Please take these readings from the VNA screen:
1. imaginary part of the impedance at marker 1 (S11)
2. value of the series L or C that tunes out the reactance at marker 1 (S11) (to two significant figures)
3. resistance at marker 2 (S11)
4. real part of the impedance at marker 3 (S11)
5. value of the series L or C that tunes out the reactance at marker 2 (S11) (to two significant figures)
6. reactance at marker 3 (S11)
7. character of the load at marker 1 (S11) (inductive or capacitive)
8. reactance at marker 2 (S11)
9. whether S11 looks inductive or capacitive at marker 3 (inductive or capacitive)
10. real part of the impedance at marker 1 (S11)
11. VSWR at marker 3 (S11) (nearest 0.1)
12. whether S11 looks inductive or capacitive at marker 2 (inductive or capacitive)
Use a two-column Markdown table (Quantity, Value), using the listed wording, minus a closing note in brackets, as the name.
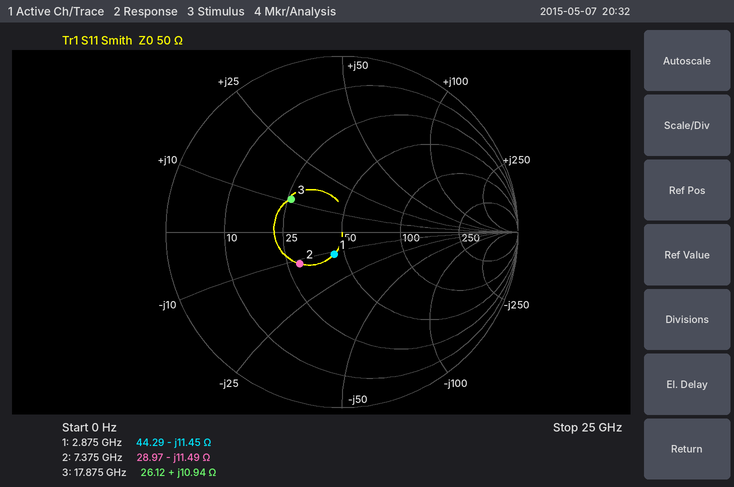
| Quantity | Value |
|---|---|
| imaginary part of the impedance at marker 1 | -11.45 Ω |
| value of the series L or C that tunes out the reactance at marker 1 (S11) | 630 pH |
| resistance at marker 2 | 28.97 Ω |
| real part of the impedance at marker 3 | 26.12 Ω |
| value of the series L or C that tunes out the reactance at marker 2 (S11) | 250 pH |
| reactance at marker 3 | +10.94 Ω |
| character of the load at marker 1 (S11) | capacitive |
| reactance at marker 2 | -11.49 Ω |
| whether S11 looks inductive or capacitive at marker 3 | inductive |
| real part of the impedance at marker 1 | 44.29 Ω |
| VSWR at marker 3 (S11) | 2.0 |
| whether S11 looks inductive or capacitive at marker 2 | capacitive |
